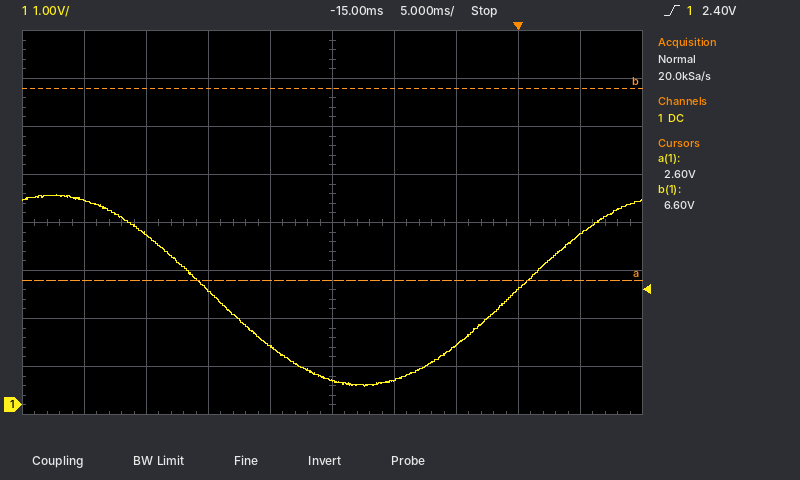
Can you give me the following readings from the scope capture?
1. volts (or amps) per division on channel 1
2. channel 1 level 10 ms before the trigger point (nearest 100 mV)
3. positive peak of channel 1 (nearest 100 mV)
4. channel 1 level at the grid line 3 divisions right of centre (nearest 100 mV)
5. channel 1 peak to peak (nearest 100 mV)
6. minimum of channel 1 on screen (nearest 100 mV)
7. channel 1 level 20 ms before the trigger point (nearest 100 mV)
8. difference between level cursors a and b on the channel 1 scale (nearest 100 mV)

1 V
500 mV
4.4 V
2.4 V
4.0 V
400 mV
1.2 V
4.0 V
